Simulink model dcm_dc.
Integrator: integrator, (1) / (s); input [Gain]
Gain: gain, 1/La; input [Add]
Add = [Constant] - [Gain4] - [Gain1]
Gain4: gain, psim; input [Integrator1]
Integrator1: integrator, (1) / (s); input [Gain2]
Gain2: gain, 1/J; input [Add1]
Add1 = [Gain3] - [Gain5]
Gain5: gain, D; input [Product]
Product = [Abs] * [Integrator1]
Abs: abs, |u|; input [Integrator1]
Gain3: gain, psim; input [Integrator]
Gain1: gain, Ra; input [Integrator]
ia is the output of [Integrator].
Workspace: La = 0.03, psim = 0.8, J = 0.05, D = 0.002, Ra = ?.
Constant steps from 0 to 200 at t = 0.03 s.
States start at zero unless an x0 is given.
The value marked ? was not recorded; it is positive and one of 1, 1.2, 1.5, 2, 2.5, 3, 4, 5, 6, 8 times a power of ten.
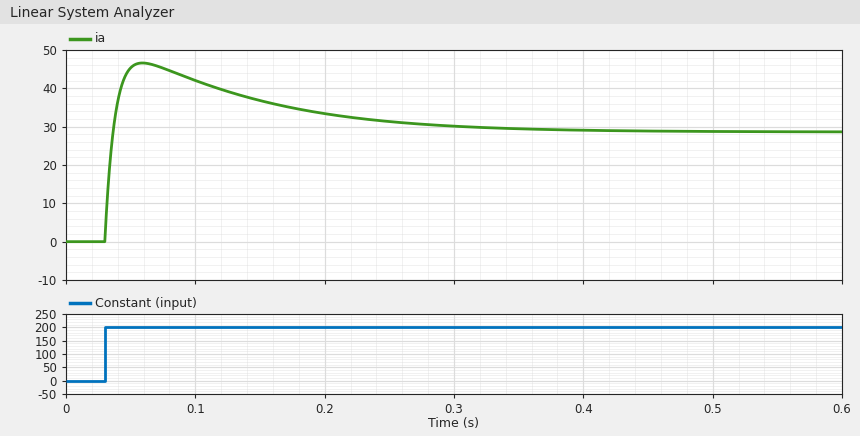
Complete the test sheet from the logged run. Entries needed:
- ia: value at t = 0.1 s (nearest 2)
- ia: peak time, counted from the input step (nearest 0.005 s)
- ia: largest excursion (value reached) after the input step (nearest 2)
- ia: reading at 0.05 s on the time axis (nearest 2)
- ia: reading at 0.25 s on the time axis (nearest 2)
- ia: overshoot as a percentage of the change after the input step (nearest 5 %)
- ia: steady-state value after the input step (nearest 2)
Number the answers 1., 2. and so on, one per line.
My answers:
1. 42
2. 0.030 s
3. 46
4. 46
5. 32
6. 65 %
7. 28
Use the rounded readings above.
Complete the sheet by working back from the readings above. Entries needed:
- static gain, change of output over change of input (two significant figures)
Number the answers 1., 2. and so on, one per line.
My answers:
1. 0.14
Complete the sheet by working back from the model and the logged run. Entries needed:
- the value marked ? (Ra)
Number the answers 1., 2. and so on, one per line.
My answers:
1. 4
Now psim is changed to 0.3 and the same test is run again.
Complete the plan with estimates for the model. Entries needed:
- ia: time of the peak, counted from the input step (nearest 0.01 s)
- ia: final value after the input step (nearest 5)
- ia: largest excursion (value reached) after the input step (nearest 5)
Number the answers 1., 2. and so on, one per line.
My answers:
1. 0.04 s
2. 45
3. 50
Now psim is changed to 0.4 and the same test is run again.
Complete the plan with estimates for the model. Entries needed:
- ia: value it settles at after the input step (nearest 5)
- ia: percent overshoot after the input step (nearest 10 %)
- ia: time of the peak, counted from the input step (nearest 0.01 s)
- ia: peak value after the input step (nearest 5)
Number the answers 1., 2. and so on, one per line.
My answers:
1. 40
2. 20 %
3. 0.04 s
4. 50
